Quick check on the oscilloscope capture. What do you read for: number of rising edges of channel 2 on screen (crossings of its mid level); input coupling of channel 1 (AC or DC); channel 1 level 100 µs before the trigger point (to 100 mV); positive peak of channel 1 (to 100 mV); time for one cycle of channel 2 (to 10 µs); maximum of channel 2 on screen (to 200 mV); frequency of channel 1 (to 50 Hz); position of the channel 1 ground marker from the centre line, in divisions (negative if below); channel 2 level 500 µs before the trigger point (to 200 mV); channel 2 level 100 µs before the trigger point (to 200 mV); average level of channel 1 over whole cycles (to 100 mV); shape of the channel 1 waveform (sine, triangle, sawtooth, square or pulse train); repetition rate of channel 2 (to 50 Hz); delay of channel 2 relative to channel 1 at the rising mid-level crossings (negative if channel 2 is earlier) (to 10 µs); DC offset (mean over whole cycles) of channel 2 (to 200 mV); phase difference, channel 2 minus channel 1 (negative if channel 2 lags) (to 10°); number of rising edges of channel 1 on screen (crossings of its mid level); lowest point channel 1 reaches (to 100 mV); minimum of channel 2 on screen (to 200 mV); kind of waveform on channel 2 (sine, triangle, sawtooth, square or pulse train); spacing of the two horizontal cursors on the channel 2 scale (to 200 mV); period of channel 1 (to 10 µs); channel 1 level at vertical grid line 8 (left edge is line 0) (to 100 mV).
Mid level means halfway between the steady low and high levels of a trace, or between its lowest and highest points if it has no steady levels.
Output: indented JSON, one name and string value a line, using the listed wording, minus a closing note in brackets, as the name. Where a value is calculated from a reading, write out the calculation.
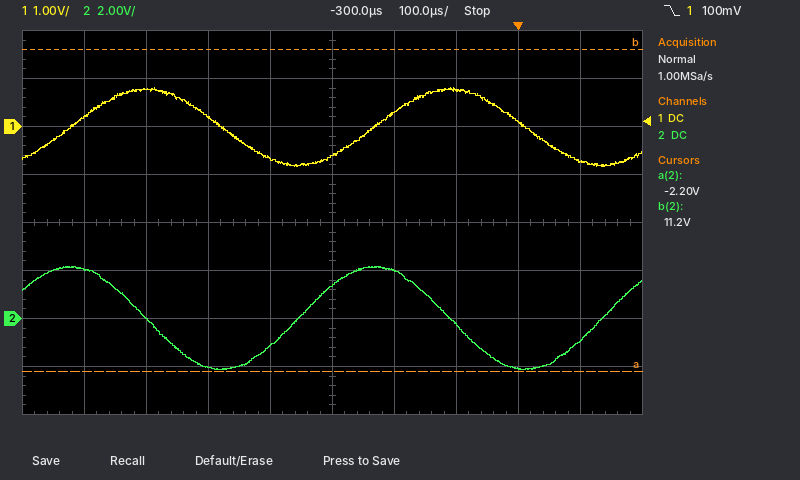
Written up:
{
  "number of rising edges of channel 2 on screen": "2",
  "input coupling of channel 1": "DC",
  "channel 1 level 100 µs before the trigger point": "800 mV",
  "positive peak of channel 1": "800 mV",
  "time for one cycle of channel 2": "490 µs",
  "maximum of channel 2 on screen": "2.2 V",
  "frequency of channel 1": "1 / 490 µs ≈ 2.04 kHz, so 2.05 kHz to the nearest 50 Hz",
  "position of the channel 1 ground marker from the centre line, in divisions": "+2.0 div",
  "channel 2 level 500 µs before the trigger point": "-2.0 V",
  "channel 2 level 100 µs before the trigger point": "-200 mV",
  "average level of channel 1 over whole cycles": "(800 mV + (-800 mV)) / 2 ≈ 0.0 V",
  "shape of the channel 1 waveform": "sine",
  "repetition rate of channel 2": "1 / 490 µs ≈ 2.04 kHz, so 2.05 kHz to the nearest 50 Hz",
  "delay of channel 2 relative to channel 1 at the rising mid-level crossings (negative if channel 2 is earlier)": "-120 µs",
  "DC offset (mean over whole cycles) of channel 2": "(2.2 V + (-2.2 V)) / 2 ≈ 0.0 V",
  "phase difference, channel 2 minus channel 1 (negative if channel 2 lags)": "−360° × (-120 µs) / 490 µs ≈ +88.2°, so +90° to the nearest 10°",
  "number of rising edges of channel 1 on screen": "2",
  "lowest point channel 1 reaches": "-800 mV",
  "minimum of channel 2 on screen": "-2.2 V",
  "kind of waveform on channel 2": "sine",
  "spacing of the two horizontal cursors on the channel 2 scale": "13.4 V",
  "period of channel 1": "490 µs",
  "channel 1 level at vertical grid line 8 (left edge is line 0)": "100 mV"
}
